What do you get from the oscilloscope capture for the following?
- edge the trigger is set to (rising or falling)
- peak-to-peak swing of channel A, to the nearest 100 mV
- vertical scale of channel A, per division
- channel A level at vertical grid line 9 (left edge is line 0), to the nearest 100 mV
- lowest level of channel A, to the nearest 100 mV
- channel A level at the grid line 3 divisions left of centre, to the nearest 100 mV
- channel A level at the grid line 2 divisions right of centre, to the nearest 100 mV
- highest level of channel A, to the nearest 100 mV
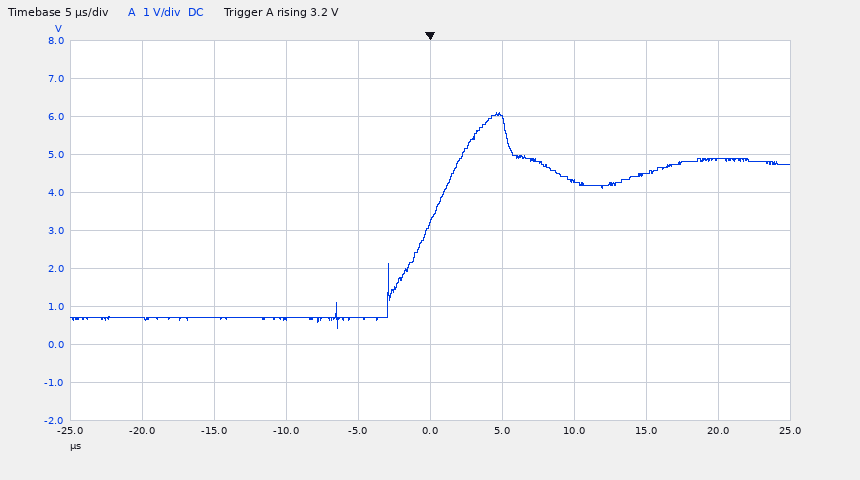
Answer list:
rising
5.7 V
1 V
4.9 V
400 mV
700 mV
4.3 V
6.1 V
